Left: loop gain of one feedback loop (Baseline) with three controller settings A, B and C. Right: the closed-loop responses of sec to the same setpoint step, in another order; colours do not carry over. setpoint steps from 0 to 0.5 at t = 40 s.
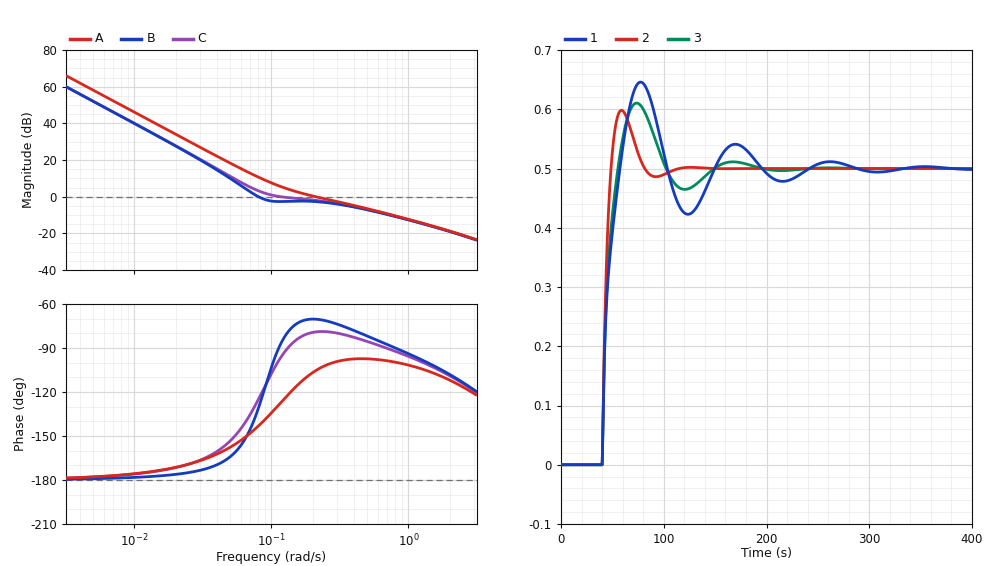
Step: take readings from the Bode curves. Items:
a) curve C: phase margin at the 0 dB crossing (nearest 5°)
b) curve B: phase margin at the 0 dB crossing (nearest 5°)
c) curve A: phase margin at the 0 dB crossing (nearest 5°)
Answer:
85°
50°
75°
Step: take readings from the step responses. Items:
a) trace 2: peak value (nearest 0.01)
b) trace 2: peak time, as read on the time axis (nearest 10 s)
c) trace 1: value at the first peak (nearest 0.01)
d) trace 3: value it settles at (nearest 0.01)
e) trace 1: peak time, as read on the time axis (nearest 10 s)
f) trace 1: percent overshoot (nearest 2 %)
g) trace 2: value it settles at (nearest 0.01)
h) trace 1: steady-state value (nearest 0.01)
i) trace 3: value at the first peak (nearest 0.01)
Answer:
0.60
60 s
0.65
0.50
80 s
30 %
0.50
0.50
0.61
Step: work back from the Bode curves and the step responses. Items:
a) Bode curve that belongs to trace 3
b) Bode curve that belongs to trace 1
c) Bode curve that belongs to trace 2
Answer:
C
B
A
